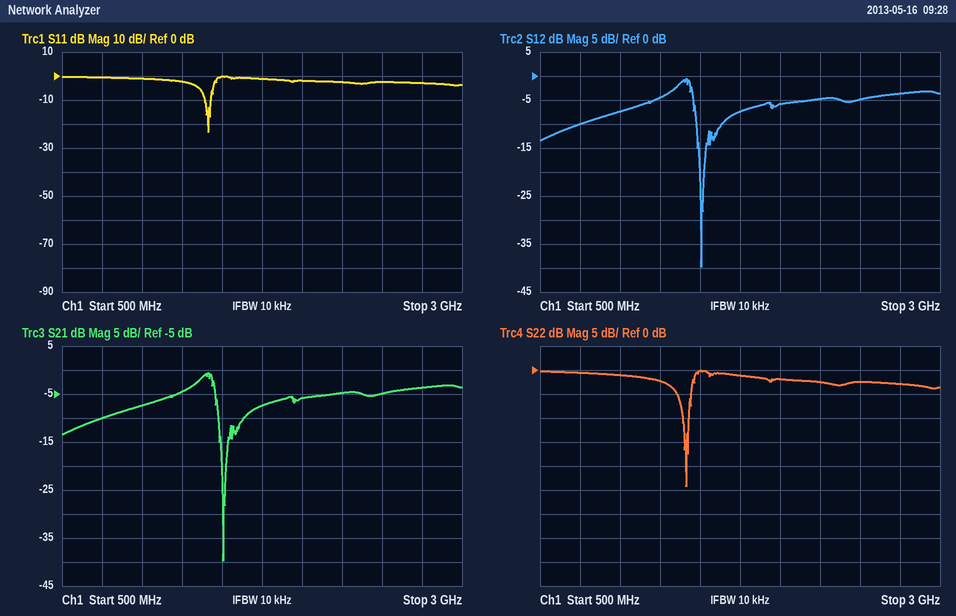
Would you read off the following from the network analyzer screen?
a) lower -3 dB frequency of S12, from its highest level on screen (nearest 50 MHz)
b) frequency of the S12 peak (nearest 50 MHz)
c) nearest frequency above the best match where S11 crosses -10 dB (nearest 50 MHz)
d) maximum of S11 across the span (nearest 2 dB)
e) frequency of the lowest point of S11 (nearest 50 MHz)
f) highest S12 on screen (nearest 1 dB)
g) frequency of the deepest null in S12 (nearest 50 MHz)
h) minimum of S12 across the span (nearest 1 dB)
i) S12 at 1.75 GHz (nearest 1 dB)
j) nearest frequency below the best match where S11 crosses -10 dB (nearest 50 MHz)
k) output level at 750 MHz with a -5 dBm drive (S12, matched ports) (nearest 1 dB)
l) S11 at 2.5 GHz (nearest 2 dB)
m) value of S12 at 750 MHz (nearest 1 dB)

1.30 GHz
1.40 GHz
1.45 GHz
0 dB
1.40 GHz
-1 dB
1.50 GHz
-40 dB
-7 dB
1.40 GHz
-15 dBm
-2 dB
-10 dB
